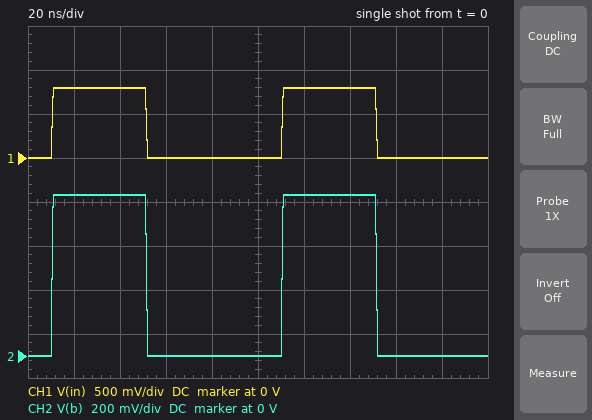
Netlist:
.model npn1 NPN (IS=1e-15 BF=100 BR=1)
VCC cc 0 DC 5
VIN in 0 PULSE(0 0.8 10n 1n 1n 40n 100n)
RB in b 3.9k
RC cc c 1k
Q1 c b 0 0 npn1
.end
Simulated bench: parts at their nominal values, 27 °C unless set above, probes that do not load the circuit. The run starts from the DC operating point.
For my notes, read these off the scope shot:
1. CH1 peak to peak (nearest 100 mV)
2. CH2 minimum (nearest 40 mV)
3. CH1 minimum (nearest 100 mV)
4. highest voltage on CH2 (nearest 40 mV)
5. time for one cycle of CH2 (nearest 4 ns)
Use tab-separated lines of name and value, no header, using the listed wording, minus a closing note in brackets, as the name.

CH1 peak to peak	800 mV
CH2 minimum	0 V
CH1 minimum	0 V
highest voltage on CH2	720 mV
time for one cycle of CH2	100 ns
